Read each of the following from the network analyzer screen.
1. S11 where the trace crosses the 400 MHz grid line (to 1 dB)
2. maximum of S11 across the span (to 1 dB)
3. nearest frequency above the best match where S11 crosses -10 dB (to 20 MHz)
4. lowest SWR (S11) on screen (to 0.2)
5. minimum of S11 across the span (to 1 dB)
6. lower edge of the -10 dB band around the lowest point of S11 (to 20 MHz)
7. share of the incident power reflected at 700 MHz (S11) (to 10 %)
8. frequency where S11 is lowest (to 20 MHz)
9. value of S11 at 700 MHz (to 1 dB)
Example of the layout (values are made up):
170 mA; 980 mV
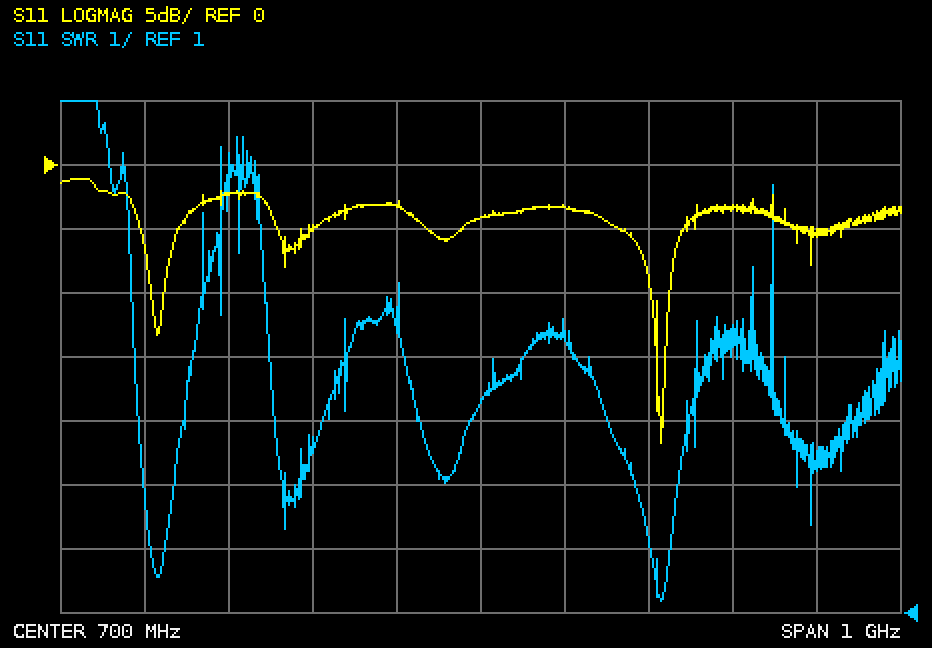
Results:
-2 dB; -1 dB; 920 MHz; 1.2; -22 dB; 900 MHz; 40 %; 920 MHz; -4 dB
